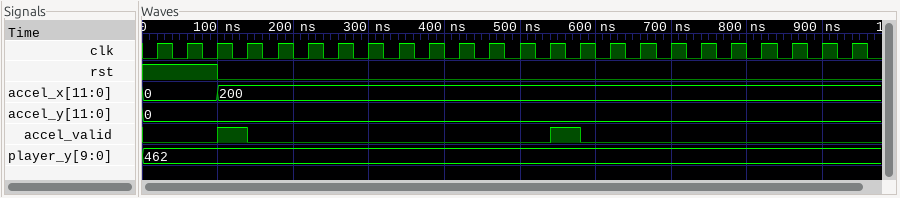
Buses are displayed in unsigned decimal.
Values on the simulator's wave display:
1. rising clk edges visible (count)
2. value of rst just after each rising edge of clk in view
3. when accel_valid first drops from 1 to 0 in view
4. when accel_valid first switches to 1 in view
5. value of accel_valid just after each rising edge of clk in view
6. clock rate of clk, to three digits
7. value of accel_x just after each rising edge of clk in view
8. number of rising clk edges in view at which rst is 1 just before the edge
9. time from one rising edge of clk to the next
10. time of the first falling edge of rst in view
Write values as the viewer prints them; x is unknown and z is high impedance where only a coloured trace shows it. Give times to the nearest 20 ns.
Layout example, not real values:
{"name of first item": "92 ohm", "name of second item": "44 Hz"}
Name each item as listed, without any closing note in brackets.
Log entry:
{"rising clk edges visible": "24", "value of rst just after each rising edge of clk in view": "1 1 0 0 0 0 0 0 0 0 0 0 0 0 0 0 0 0 0 0 0 0 0 0", "when accel_valid first drops from 1 to 0 in view": "140 ns", "when accel_valid first switches to 1 in view": "100 ns", "value of accel_valid just after each rising edge of clk in view": "0 0 1 0 0 0 0 0 0 0 0 0 0 1 0 0 0 0 0 0 0 0 0 0", "clock rate of clk, to three digits": "25.0 MHz", "value of accel_x just after each rising edge of clk in view": "0, 0, 200, 200, 200, 200, 200, 200, 200, 200, 200, 200, 200, 200, 200, 200, 200, 200, 200, 200, 200, 200, 200, 200", "number of rising clk edges in view at which rst is 1 just before the edge": "3", "time from one rising edge of clk to the next": "40 ns", "time of the first falling edge of rst in view": "100 ns"}
